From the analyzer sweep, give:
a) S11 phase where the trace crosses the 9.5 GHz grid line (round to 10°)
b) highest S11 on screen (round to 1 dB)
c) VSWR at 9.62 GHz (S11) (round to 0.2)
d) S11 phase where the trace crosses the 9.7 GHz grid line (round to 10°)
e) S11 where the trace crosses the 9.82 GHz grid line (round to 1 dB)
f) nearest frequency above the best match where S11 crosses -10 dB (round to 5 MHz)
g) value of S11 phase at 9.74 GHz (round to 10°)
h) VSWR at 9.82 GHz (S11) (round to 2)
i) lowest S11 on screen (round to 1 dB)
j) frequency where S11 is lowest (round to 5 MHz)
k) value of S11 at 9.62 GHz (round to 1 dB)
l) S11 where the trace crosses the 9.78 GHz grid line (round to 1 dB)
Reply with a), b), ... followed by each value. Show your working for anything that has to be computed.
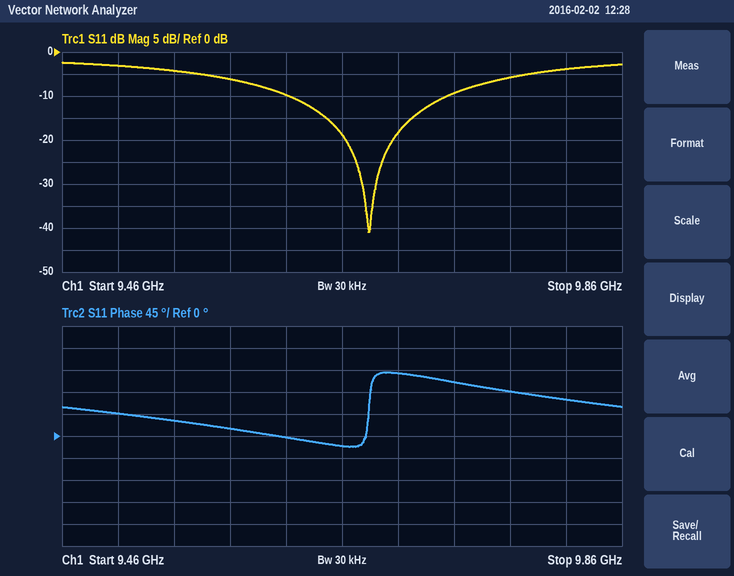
a) 50°
b) -2 dB
c) |Γ| = 10^(-10/20) = 0.3162; VSWR = (1 + 0.3162)/(1 − 0.3162) ≈ 1.92, so 2.0 to the nearest 0.2
d) 130°
e) -4 dB
f) 9.735 GHz
g) 110°
h) |Γ| = 10^(-4/20) = 0.6310; VSWR = (1 + 0.6310)/(1 − 0.6310) ≈ 4
i) -41 dB
j) 9.680 GHz
k) -10 dB
l) -6 dB
